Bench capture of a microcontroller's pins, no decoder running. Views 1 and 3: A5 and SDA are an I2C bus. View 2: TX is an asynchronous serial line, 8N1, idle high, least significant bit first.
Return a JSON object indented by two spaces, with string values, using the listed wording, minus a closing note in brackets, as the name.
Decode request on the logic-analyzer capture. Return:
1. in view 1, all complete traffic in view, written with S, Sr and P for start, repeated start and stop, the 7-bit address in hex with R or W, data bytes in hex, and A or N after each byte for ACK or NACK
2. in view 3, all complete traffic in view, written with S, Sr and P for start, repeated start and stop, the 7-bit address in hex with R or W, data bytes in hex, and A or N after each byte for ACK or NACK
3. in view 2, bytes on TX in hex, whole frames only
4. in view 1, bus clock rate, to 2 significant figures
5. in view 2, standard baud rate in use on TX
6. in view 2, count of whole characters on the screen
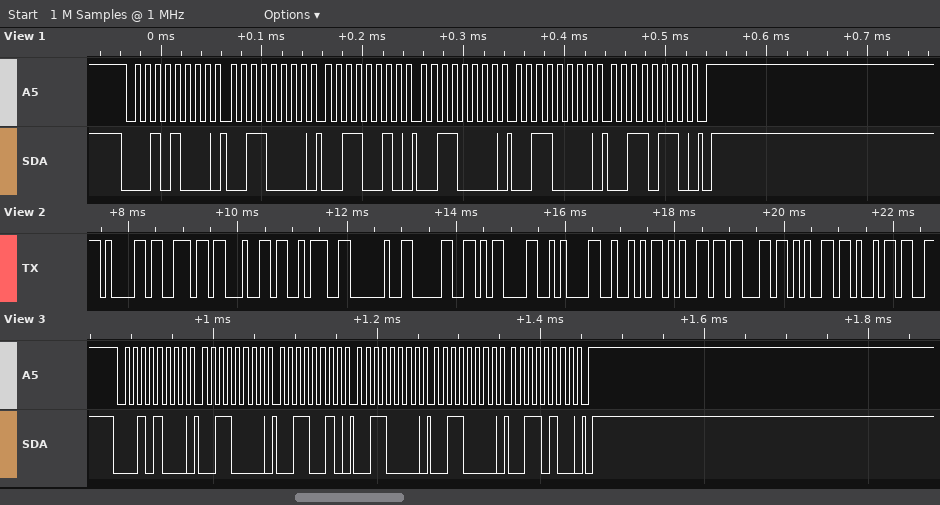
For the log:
{
  "in view 1, all complete traffic in view, written with S, Sr and P for start, repeated start and stop, the 7-bit address in hex with R or W, data bytes in hex, and A or N after each byte for ACK or NACK": "S 14W A 30 A 32 A 30 A 30 A 36 A P",
  "in view 3, all complete traffic in view, written with S, Sr and P for start, repeated start and stop, the 7-bit address in hex with R or W, data bytes in hex, and A or N after each byte for ACK or NACK": "S 14W A 30 A 32 A 30 A 30 A 34 A P",
  "in view 2, bytes on TX in hex, whole frames only": "0x61 0x6E 0x64 0x3A 0x20 0x30 0x0D 0x0A 0x52 0x65 0x63 0x65 0x69",
  "in view 1, bus clock rate, to 2 significant figures": "100 kHz",
  "in view 2, standard baud rate in use on TX": "9600 baud",
  "in view 2, count of whole characters on the screen": "13"
}
